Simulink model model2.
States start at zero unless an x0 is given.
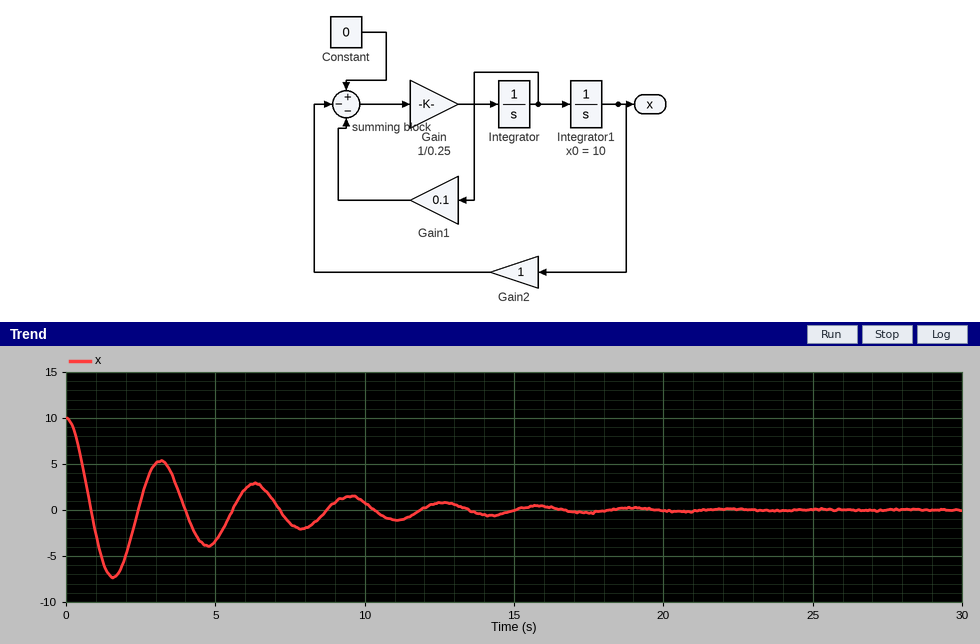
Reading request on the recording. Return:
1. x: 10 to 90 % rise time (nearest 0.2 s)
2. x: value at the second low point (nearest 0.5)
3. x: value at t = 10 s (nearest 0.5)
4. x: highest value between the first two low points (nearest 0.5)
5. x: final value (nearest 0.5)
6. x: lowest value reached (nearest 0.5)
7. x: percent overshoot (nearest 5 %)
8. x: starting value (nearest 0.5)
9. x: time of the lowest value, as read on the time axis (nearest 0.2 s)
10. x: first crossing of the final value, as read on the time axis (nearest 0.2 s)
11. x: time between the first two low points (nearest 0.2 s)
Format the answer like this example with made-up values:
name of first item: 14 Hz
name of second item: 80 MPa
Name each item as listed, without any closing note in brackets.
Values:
x: 10 to 90 % rise time: 0.6 s
x: value at the second low point: -4.0
x: value at t = 10 s: 1.0
x: highest value between the first two low points: 5.5
x: final value: 0.0
x: lowest value reached: -7.5
x: percent overshoot: 75 %
x: starting value: 10.0
x: time of the lowest value, as read on the time axis: 1.6 s
x: first crossing of the final value, as read on the time axis: 0.8 s
x: time between the first two low points: 3.2 s
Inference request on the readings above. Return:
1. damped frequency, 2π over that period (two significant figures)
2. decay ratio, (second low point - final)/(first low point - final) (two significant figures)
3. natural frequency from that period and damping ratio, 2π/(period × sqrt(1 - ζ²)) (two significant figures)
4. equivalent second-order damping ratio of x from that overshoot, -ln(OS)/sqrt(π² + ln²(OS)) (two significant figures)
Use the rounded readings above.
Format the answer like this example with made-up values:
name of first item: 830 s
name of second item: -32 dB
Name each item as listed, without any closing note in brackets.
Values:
damped frequency, 2π over that period: 2.0 rad/s
decay ratio, (second low point - final)/(first low point - final): 0.53
natural frequency from that period and damping ratio, 2π/(period × sqrt(1 - ζ²)): 2.0 rad/s
equivalent second-order damping ratio of x from that overshoot, -ln(OS)/sqrt(π² + ln²(OS)): 0.091
